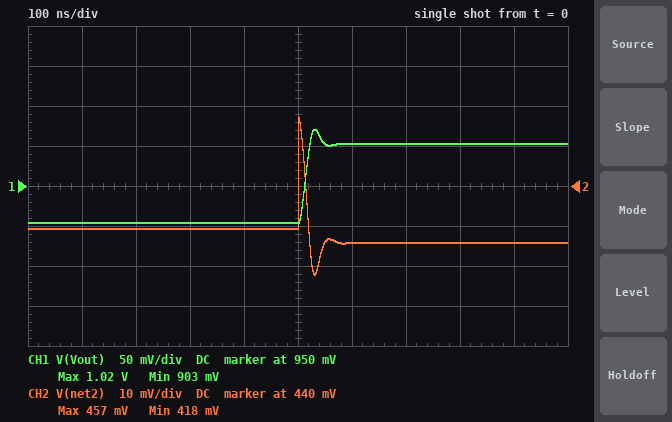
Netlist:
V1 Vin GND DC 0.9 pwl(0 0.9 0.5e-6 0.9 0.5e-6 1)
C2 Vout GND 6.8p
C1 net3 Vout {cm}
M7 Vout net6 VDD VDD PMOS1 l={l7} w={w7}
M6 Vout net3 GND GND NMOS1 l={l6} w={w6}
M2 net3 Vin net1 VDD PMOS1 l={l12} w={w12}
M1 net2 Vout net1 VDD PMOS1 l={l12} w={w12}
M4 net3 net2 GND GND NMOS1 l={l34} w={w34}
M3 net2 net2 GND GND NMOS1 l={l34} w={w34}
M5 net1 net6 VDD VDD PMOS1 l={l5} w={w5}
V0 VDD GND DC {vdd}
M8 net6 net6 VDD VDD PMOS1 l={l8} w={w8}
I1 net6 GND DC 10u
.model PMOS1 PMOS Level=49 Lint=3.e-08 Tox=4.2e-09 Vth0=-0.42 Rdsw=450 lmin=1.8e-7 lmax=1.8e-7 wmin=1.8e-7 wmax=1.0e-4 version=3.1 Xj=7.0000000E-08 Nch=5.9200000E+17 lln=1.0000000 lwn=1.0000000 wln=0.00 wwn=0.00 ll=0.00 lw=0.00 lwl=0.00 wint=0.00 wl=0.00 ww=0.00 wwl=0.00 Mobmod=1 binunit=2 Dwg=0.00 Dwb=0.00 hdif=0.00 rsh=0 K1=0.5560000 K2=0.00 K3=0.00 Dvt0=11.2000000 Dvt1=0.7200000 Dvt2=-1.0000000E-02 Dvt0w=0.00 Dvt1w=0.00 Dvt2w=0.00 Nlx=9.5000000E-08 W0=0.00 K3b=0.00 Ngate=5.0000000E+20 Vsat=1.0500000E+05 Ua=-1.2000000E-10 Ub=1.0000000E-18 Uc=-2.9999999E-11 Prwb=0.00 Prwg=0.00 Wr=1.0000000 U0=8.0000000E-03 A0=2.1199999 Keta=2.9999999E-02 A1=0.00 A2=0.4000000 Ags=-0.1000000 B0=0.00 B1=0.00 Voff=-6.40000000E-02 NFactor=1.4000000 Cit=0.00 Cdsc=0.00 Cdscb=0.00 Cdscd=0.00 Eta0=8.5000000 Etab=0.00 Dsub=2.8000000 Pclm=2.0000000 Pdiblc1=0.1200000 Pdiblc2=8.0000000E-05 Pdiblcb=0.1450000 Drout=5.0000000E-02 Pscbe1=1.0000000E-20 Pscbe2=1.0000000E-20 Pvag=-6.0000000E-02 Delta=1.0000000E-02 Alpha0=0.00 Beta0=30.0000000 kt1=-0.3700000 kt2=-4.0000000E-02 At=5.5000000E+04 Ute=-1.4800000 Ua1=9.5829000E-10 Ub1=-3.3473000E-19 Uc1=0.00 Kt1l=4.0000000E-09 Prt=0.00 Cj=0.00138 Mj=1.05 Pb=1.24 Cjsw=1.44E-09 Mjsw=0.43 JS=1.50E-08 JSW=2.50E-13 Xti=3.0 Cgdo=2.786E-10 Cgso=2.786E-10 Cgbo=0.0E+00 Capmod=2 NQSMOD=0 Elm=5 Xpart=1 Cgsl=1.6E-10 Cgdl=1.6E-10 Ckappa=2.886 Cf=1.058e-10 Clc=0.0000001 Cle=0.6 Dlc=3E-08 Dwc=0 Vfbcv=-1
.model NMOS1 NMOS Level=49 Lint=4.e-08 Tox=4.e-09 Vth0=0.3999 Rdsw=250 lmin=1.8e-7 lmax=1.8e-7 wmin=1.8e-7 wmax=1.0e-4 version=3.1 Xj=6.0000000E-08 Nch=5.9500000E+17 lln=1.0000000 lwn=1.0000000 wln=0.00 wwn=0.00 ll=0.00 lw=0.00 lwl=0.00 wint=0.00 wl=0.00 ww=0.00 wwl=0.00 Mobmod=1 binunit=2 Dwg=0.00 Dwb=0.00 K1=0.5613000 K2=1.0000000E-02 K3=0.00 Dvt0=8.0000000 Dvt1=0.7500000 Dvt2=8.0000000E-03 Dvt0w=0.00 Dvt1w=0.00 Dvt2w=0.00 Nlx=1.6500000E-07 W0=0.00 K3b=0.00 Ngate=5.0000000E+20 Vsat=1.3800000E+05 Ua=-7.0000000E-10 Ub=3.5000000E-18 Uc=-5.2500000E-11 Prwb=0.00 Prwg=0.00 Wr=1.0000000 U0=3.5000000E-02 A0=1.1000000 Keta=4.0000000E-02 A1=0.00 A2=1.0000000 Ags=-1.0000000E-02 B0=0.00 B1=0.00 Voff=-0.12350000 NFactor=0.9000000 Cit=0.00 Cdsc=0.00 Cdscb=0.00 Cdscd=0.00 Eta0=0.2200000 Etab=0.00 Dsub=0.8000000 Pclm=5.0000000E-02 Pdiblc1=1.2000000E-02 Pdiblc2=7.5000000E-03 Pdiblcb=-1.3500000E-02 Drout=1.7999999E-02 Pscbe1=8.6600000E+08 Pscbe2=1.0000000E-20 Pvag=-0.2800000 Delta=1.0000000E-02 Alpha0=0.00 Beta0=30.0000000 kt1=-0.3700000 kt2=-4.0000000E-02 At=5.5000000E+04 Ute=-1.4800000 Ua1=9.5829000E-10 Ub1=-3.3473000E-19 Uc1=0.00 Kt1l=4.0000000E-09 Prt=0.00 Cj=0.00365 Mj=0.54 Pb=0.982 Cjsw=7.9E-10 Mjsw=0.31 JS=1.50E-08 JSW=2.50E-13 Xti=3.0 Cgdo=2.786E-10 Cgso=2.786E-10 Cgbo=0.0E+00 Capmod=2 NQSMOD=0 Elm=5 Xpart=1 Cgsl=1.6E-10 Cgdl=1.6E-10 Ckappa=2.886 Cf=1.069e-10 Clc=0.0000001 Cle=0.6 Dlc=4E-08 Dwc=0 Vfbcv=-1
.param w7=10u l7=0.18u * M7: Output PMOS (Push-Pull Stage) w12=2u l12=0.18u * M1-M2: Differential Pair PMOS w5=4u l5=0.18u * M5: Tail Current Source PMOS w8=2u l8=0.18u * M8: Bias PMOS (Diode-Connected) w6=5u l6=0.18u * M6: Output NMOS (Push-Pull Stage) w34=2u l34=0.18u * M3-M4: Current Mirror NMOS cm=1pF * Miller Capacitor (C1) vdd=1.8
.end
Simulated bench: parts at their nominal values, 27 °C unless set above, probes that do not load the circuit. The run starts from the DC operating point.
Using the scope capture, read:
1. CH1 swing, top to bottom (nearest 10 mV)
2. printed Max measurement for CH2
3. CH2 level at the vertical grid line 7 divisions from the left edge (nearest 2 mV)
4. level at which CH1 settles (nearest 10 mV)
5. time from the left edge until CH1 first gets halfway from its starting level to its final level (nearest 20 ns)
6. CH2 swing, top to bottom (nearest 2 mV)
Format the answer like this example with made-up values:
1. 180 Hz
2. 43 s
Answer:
1. 120 mV
2. 457 mV
3. 426 mV
4. 1.00 V
5. 520 ns
6. 40 mV
